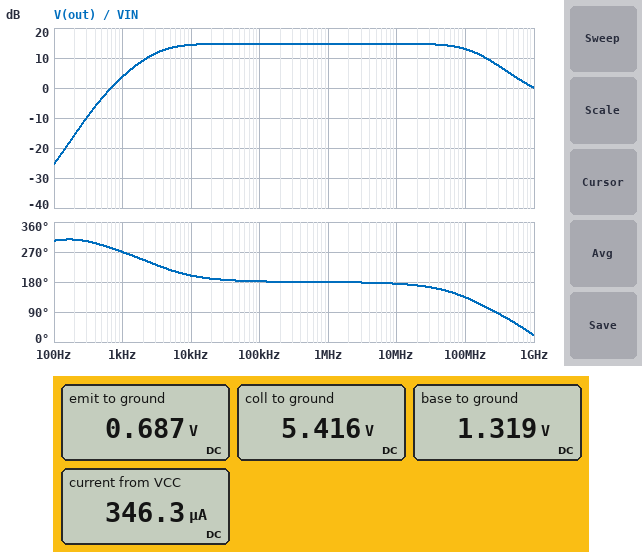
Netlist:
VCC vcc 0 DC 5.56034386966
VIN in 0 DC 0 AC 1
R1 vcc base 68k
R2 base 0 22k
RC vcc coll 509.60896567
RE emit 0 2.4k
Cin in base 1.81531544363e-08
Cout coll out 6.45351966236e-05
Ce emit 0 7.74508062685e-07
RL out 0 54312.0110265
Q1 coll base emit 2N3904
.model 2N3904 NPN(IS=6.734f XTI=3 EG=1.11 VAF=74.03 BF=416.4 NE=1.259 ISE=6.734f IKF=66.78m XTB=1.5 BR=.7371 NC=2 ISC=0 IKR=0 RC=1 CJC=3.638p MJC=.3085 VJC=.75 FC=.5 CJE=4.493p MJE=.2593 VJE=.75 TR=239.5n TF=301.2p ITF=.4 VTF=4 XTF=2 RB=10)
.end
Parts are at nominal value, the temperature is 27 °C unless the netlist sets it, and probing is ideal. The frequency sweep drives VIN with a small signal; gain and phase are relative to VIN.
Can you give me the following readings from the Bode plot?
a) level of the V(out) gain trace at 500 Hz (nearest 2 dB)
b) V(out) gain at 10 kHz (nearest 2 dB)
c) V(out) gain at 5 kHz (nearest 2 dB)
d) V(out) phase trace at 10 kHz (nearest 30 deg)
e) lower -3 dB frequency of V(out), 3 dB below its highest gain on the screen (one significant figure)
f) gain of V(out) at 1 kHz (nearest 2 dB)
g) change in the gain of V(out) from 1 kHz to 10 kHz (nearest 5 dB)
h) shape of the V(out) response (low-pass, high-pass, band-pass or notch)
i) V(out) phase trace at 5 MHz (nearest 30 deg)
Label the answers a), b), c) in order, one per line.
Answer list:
a) -4 dB
b) 14 dB
c) 14 dB
d) 210 deg
e) 3 kHz
f) 4 dB
g) 10 dB
h) band-pass
i) 180 deg
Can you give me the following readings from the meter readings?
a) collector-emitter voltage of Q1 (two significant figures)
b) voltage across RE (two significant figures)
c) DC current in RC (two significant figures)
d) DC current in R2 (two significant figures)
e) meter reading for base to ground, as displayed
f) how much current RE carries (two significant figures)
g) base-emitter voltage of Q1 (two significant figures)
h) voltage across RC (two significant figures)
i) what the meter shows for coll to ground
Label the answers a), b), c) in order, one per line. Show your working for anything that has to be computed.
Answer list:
a) 5.416 V - 687 mV = 4.7 V
b) 687 mV = 690 mV
c) (5.56 V - 5.416 V) / 509.6 Ω = 280 µA
d) (1.319 V) / 22 kΩ = 60 µA
e) 1.319 V
f) (687 mV) / 2.4 kΩ = 290 µA
g) 1.319 V - 687 mV = 630 mV
h) 5.56 V - 5.416 V = 140 mV
i) 5.416 V
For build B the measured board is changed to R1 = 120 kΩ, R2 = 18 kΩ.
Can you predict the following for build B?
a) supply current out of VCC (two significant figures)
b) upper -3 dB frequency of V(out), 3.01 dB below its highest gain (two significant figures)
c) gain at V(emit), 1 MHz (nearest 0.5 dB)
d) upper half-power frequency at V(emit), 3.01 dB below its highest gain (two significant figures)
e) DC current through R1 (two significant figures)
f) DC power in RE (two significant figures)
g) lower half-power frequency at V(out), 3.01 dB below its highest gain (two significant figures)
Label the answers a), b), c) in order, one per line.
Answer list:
a) 93 µA
b) 2.1 GHz
c) -67.5 dB
d) 1.4 kHz
e) 40 µA
f) 6.9 µW
g) 1.0 kHz
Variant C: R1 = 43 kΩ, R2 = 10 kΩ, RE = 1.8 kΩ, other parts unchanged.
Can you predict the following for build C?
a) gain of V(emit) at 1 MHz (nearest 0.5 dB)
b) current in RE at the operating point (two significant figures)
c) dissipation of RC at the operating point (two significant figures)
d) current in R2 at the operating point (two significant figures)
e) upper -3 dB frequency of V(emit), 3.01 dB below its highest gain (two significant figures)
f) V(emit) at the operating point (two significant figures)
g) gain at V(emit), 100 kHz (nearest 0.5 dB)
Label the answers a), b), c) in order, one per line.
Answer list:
a) -55.0 dB
b) 230 µA
c) 26 µW
d) 100 µA
e) 4.1 kHz
f) 410 mV
g) -35.0 dB
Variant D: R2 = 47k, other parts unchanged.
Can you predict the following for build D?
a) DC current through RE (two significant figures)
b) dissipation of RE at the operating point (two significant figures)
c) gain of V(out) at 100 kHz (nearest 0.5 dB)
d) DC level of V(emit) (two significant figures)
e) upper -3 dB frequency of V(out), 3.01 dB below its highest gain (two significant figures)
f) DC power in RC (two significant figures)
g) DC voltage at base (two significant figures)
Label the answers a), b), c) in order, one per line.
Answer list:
a) 620 µA
b) 920 µW
c) 21.5 dB
d) 1.5 V
e) 110 MHz
f) 190 µW
g) 2.1 V
